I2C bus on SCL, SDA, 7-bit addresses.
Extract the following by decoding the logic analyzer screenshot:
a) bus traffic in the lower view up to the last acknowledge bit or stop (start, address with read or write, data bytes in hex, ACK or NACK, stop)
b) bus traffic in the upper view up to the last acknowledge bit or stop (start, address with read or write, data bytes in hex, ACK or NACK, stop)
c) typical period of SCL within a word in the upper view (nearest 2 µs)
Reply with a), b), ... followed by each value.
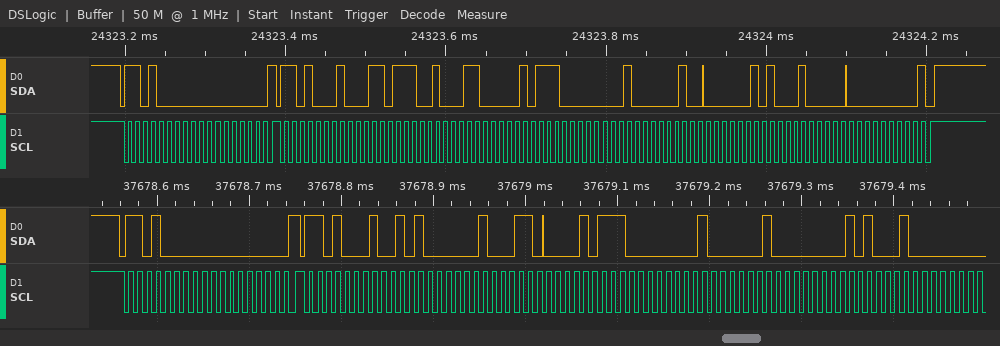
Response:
a) start, address 68 write ACK, 00 ACK, repeated start, address 68 read ACK, 50 ACK, 46 ACK, 17 ACK, 01 ACK, 04 ACK, 05 ACK, 20 ACK
b) start, address 68 write ACK, 00 ACK, repeated start, address 68 read ACK, 37 ACK, 46 ACK, 17 ACK, 01 ACK, 04 ACK, 05 ACK, 20 ACK, 00 NACK, stop
c) 10 µs
